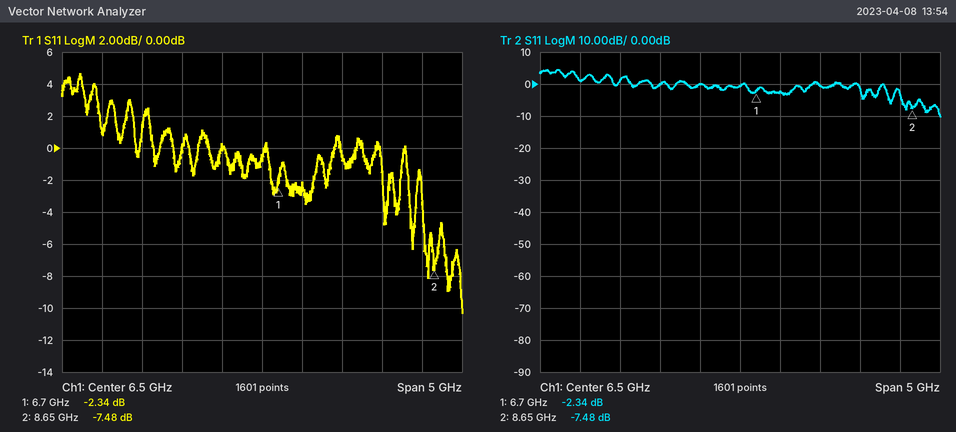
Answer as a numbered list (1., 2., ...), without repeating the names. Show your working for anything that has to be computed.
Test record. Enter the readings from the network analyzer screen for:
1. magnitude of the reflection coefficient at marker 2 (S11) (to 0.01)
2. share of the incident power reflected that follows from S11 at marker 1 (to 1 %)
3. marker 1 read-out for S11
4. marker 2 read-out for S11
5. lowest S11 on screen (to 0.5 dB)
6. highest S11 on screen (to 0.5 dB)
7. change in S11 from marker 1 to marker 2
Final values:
1. 10^(-7.48/20) ≈ 0.42
2. 10^(-2.34/10) ≈ 58 %
3. -2.34 dB
4. -7.48 dB
5. -10.5 dB
6. 4.5 dB
7. -7.48 − (-2.34) = -5.14 dB
